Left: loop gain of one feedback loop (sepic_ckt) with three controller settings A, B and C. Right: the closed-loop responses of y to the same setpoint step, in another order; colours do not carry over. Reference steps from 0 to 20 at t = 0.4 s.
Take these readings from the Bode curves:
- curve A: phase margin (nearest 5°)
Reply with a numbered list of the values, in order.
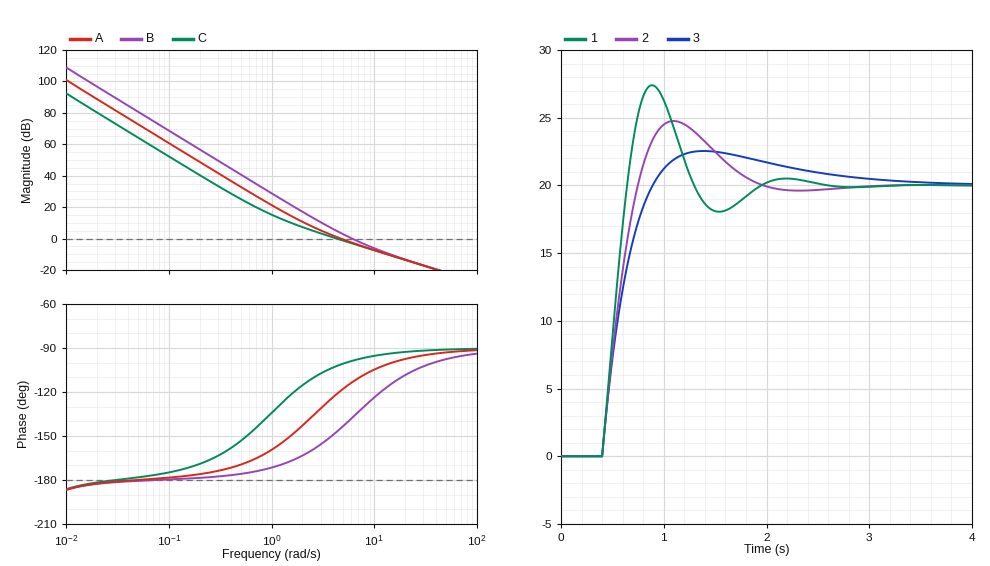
1. 60°
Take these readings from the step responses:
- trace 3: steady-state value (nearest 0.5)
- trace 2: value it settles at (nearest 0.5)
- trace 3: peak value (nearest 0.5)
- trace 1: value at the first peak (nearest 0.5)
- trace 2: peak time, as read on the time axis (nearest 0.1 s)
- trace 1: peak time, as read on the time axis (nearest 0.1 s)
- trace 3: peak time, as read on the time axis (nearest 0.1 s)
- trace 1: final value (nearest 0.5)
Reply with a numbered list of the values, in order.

1. 20.0
2. 20.0
3. 22.5
4. 27.5
5. 1.1 s
6. 0.9 s
7. 1.4 s
8. 20.0
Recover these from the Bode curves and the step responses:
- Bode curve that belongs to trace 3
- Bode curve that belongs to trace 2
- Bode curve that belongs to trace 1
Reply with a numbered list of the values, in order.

1. C
2. A
3. B
